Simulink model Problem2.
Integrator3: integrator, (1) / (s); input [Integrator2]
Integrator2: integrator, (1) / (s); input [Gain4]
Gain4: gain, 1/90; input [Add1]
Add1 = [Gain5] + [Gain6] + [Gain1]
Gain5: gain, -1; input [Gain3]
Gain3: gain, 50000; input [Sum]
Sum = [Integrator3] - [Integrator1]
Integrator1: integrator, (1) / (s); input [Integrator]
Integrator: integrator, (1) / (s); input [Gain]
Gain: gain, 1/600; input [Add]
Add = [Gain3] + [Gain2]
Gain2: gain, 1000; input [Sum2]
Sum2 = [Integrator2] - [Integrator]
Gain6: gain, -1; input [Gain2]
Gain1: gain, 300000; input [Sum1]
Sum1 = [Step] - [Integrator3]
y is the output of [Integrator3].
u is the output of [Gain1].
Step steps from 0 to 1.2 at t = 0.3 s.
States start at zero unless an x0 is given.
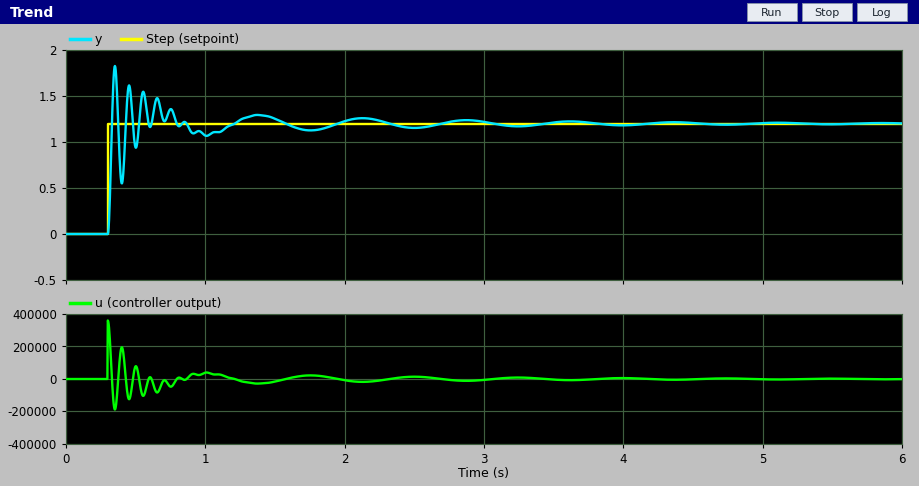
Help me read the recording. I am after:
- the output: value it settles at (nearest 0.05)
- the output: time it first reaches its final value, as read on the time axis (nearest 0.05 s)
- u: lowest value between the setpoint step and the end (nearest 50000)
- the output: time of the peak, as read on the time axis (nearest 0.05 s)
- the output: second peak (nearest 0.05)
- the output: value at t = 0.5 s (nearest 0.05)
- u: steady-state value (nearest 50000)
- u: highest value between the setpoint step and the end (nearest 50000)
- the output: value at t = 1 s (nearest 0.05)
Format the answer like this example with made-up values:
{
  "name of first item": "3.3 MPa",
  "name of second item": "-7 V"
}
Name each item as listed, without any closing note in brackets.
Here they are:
{
  "the output: value it settles at": "1.20",
  "the output: time it first reaches its final value, as read on the time axis": "0.35 s",
  "u: lowest value between the setpoint step and the end": "-200000",
  "the output: time of the peak, as read on the time axis": "0.35 s",
  "the output: second peak": "1.60",
  "the output: value at t = 0.5 s": "0.95",
  "u: steady-state value": "0",
  "u: highest value between the setpoint step and the end": "350000",
  "the output: value at t = 1 s": "1.05"
}
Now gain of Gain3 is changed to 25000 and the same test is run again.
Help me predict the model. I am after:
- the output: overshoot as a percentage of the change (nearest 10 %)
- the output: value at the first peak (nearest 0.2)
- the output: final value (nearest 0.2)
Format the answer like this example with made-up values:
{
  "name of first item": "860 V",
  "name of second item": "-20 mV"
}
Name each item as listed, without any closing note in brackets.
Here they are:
{
  "the output: overshoot as a percentage of the change": "60 %",
  "the output: value at the first peak": "2.0",
  "the output: final value": "1.2"
}
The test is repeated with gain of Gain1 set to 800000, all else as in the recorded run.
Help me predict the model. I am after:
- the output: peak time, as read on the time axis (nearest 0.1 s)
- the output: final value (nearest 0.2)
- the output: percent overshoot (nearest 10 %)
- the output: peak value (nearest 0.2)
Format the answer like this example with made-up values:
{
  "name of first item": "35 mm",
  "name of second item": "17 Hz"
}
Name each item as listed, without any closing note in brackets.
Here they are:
{
  "the output: peak time, as read on the time axis": "0.3 s",
  "the output: final value": "1.2",
  "the output: percent overshoot": "70 %",
  "the output: peak value": "2.0"
}
